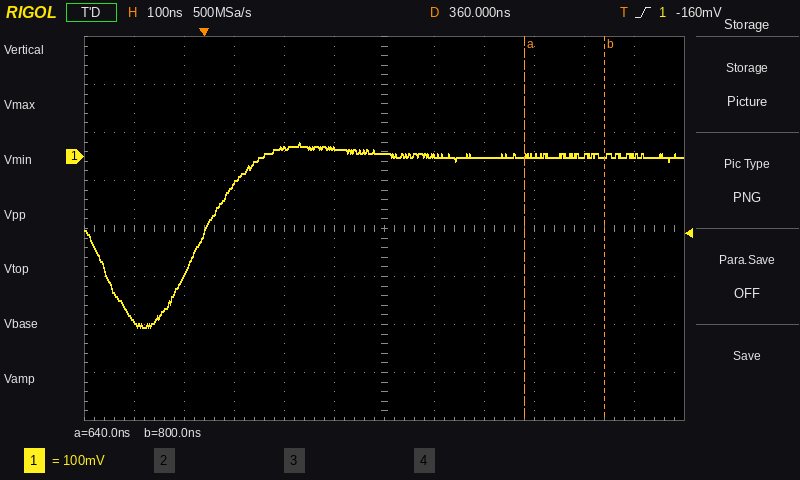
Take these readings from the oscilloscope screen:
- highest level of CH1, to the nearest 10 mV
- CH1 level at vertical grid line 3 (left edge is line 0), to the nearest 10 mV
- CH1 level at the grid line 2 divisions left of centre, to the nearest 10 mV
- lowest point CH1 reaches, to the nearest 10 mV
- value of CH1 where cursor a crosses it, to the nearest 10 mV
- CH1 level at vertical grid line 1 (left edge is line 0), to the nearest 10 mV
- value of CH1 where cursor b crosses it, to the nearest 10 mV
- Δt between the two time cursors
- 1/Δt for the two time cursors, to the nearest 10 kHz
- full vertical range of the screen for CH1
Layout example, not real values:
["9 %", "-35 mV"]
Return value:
["30 mV", "-60 mV", "20 mV", "-360 mV", "0 mV", "-340 mV", "0 mV", "160 ns", "6.25 MHz", "800 mV"]
